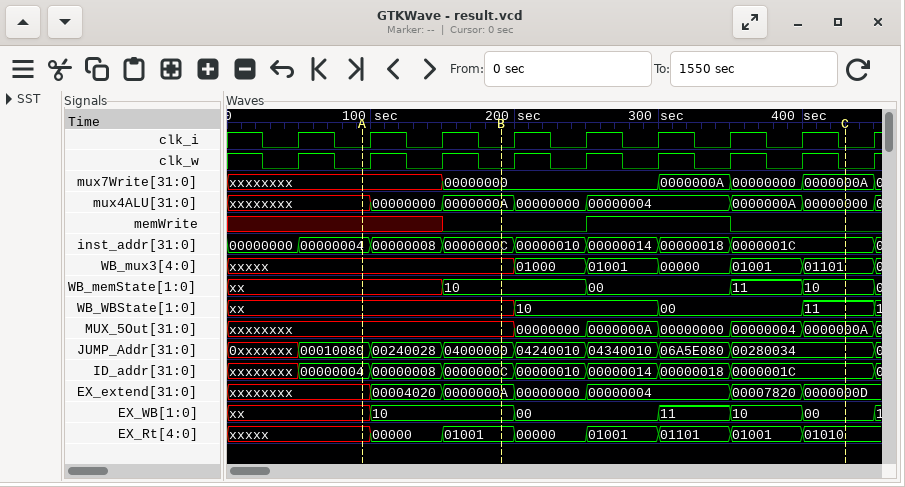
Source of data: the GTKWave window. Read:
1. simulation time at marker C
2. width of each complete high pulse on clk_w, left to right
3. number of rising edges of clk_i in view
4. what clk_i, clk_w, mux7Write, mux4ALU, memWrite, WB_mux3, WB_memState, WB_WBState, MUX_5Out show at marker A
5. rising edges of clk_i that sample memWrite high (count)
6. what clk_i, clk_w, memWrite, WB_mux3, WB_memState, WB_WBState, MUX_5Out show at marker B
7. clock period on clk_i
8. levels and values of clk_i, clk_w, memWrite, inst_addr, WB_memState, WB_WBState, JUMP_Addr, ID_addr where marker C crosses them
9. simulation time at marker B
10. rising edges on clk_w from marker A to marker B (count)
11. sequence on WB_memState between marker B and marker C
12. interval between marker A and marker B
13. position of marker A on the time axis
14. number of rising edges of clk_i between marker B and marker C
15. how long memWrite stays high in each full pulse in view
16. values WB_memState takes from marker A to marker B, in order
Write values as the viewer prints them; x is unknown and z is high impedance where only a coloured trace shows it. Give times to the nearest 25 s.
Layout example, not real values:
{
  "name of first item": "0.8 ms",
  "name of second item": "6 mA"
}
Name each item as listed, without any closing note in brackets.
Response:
{
  "simulation time at marker C": "425 s",
  "width of each complete high pulse on clk_w, left to right": "25 s, 25 s, 25 s, 25 s, 25 s, 25 s, 25 s, 25 s",
  "number of rising edges of clk_i in view": "9",
  "what clk_i, clk_w, mux7Write, mux4ALU, memWrite, WB_mux3, WB_memState, WB_WBState, MUX_5Out show at marker A": "clk_i=0, clk_w=0, mux7Write=xxxxxxxx, mux4ALU=xxxxxxxx, memWrite=x, WB_mux3=xxxxx, WB_memState=xx, WB_WBState=xx, MUX_5Out=xxxxxxxx",
  "rising edges of clk_i that sample memWrite high": "2",
  "what clk_i, clk_w, memWrite, WB_mux3, WB_memState, WB_WBState, MUX_5Out show at marker B": "clk_i=0, clk_w=0, memWrite=0, WB_mux3=xxxxx, WB_memState=10, WB_WBState=xx, MUX_5Out=xxxxxxxx",
  "clock period on clk_i": "50 s",
  "levels and values of clk_i, clk_w, memWrite, inst_addr, WB_memState, WB_WBState, JUMP_Addr, ID_addr where marker C crosses them": "clk_i=0, clk_w=0, memWrite=0, inst_addr=0000001C, WB_memState=10, WB_WBState=11, JUMP_Addr=00280034, ID_addr=0000001C",
  "simulation time at marker B": "200 s",
  "rising edges on clk_w from marker A to marker B": "2",
  "sequence on WB_memState between marker B and marker C": "10, 00, 11, 10",
  "interval between marker A and marker B": "100 s",
  "position of marker A on the time axis": "100 s",
  "number of rising edges of clk_i between marker B and marker C": "5",
  "how long memWrite stays high in each full pulse in view": "100 s",
  "values WB_memState takes from marker A to marker B, in order": "xx, 10"
}
